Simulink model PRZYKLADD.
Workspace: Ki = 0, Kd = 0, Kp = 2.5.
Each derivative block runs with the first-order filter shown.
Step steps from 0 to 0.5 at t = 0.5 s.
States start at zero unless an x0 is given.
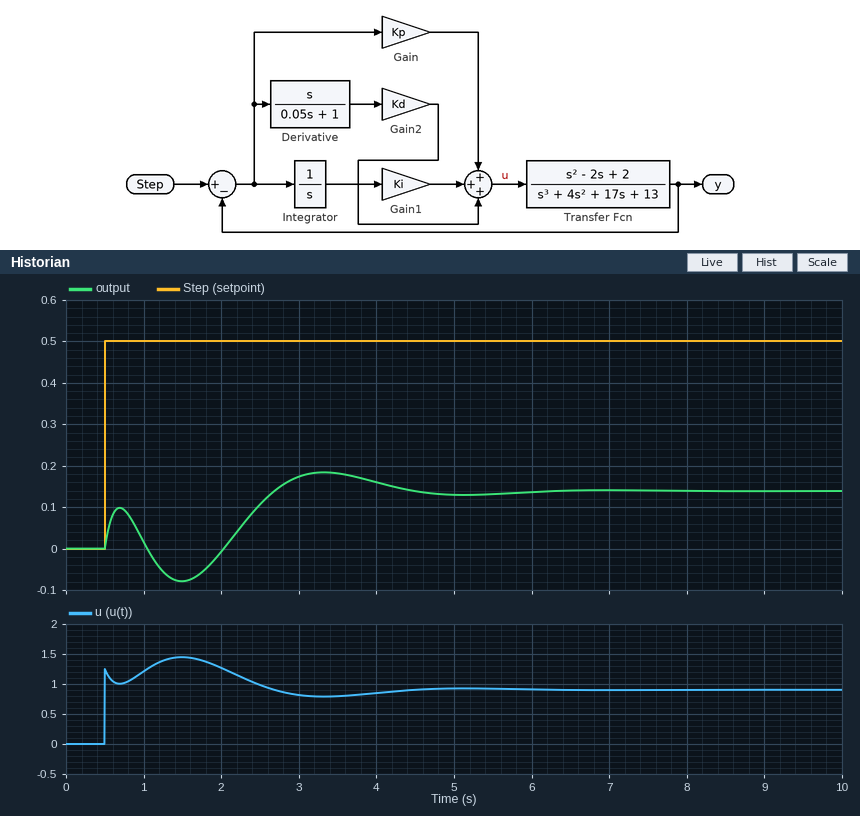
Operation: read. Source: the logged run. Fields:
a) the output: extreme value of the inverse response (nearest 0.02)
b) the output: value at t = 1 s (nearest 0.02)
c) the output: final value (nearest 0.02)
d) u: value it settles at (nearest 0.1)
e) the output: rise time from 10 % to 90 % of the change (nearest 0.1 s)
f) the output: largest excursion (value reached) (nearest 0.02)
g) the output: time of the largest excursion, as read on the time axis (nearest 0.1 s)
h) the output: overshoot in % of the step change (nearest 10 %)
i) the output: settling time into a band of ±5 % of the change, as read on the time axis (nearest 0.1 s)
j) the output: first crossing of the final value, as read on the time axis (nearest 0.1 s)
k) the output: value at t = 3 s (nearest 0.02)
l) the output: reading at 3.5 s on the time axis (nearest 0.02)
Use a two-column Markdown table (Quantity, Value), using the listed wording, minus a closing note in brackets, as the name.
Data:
| Quantity | Value |
|---|---|
| the output: extreme value of the inverse response | -0.08 |
| the output: value at t = 1 s | 0.02 |
| the output: final value | 0.14 |
| u: value it settles at | 0.9 |
| the output: rise time from 10 % to 90 % of the change | 2.1 s |
| the output: largest excursion (value reached) | 0.18 |
| the output: time of the largest excursion, as read on the time axis | 3.3 s |
| the output: overshoot in % of the step change | 30 % |
| the output: settling time into a band of ±5 % of the change, as read on the time axis | 5.6 s |
| the output: first crossing of the final value, as read on the time axis | 2.7 s |
| the output: value at t = 3 s | 0.18 |
| the output: reading at 3.5 s on the time axis | 0.18 |
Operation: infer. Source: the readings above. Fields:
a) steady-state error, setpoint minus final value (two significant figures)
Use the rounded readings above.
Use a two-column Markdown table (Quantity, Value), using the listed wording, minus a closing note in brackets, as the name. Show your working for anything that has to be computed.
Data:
| Quantity | Value |
|---|---|
| steady-state error, setpoint minus final value | 0.5 - 0.14 = 0.36 |
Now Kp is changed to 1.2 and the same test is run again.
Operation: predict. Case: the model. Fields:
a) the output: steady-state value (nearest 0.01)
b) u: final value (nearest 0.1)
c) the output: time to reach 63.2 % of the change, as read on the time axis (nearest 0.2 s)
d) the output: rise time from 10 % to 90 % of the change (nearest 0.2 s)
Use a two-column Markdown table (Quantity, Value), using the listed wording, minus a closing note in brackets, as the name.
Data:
| Quantity | Value |
|---|---|
| the output: steady-state value | 0.08 |
| u: final value | 0.5 |
| the output: time to reach 63.2 % of the change, as read on the time axis | 0.6 s |
| the output: rise time from 10 % to 90 % of the change | 2.2 s |
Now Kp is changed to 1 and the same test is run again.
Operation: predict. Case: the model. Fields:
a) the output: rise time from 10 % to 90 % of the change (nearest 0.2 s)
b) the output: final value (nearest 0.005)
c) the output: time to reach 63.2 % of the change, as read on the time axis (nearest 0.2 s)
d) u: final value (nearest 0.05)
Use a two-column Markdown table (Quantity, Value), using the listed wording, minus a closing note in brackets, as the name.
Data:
| Quantity | Value |
|---|---|
| the output: rise time from 10 % to 90 % of the change | 2.2 s |
| the output: final value | 0.065 |
| the output: time to reach 63.2 % of the change, as read on the time axis | 0.6 s |
| u: final value | 0.45 |
